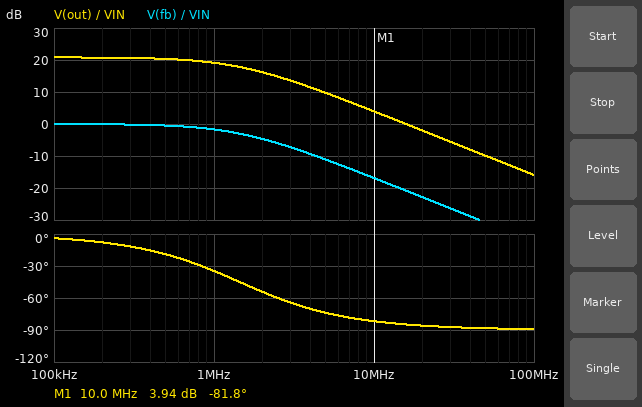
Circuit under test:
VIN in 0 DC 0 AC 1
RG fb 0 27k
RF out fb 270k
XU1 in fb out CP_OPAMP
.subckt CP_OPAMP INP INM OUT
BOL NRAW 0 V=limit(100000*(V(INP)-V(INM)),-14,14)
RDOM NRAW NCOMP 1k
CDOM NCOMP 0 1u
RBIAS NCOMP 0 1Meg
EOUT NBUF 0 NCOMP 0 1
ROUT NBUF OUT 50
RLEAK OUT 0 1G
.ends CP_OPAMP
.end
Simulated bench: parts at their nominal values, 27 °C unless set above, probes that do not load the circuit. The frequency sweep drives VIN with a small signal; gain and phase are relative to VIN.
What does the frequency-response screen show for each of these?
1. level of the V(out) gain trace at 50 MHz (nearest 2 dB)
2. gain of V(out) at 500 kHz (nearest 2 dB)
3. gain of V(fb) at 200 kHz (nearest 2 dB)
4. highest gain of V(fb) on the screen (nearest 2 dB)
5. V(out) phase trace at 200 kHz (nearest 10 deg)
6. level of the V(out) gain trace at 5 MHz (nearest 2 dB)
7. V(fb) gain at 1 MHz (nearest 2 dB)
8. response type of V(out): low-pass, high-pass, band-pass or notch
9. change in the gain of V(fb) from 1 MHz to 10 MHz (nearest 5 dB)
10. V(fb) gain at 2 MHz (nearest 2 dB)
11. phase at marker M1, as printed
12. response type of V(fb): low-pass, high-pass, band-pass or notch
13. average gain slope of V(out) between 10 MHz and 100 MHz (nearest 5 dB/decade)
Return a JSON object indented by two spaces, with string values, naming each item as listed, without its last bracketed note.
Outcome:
{
  "level of the V(out) gain trace at 50 MHz": "-10 dB",
  "gain of V(out) at 500 kHz": "20 dB",
  "gain of V(fb) at 200 kHz": "0 dB",
  "highest gain of V(fb) on the screen": "0 dB",
  "V(out) phase trace at 200 kHz": "-10 deg",
  "level of the V(out) gain trace at 5 MHz": "10 dB",
  "V(fb) gain at 1 MHz": "-2 dB",
  "response type of V(out): low-pass, high-pass, band-pass or notch": "low-pass",
  "change in the gain of V(fb) from 1 MHz to 10 MHz": "-15 dB",
  "V(fb) gain at 2 MHz": "-4 dB",
  "phase at marker M1, as printed": "-81.8 deg",
  "response type of V(fb): low-pass, high-pass, band-pass or notch": "low-pass",
  "average gain slope of V(out) between 10 MHz and 100 MHz": "-20 dB/decade"
}
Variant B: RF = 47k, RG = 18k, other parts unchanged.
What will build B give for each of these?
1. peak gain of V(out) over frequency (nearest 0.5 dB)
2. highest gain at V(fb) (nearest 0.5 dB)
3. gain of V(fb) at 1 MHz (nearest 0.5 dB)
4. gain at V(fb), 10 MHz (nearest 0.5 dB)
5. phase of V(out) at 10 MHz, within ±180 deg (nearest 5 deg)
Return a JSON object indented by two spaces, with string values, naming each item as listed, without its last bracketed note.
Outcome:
{
  "peak gain of V(out) over frequency": "11.0 dB",
  "highest gain at V(fb)": "0 dB",
  "gain of V(fb) at 1 MHz": "0 dB",
  "gain at V(fb), 10 MHz": "-8.0 dB",
  "phase of V(out) at 10 MHz, within ±180 deg": "-65 deg"
}
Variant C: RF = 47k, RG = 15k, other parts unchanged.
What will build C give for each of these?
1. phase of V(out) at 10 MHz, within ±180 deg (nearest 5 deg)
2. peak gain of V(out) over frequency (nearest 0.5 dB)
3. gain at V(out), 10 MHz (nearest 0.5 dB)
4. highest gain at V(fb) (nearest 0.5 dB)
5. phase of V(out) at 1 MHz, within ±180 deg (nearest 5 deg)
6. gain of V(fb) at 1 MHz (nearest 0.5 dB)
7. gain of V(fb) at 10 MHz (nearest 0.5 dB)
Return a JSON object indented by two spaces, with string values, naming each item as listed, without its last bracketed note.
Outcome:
{
  "phase of V(out) at 10 MHz, within ±180 deg": "-70 deg",
  "peak gain of V(out) over frequency": "12.5 dB",
  "gain at V(out), 10 MHz": "3.5 dB",
  "highest gain at V(fb)": "0 dB",
  "phase of V(out) at 1 MHz, within ±180 deg": "-15 deg",
  "gain of V(fb) at 1 MHz": "-0.5 dB",
  "gain of V(fb) at 10 MHz": "-9.0 dB"
}
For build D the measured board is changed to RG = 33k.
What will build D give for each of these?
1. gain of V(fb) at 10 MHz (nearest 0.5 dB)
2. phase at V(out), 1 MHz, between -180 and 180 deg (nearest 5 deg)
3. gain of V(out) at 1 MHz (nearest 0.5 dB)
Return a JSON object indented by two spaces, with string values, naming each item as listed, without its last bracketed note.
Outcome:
{
  "gain of V(fb) at 10 MHz": "-15.5 dB",
  "phase at V(out), 1 MHz, between -180 and 180 deg": "-30 deg",
  "gain of V(out) at 1 MHz": "18.0 dB"
}
